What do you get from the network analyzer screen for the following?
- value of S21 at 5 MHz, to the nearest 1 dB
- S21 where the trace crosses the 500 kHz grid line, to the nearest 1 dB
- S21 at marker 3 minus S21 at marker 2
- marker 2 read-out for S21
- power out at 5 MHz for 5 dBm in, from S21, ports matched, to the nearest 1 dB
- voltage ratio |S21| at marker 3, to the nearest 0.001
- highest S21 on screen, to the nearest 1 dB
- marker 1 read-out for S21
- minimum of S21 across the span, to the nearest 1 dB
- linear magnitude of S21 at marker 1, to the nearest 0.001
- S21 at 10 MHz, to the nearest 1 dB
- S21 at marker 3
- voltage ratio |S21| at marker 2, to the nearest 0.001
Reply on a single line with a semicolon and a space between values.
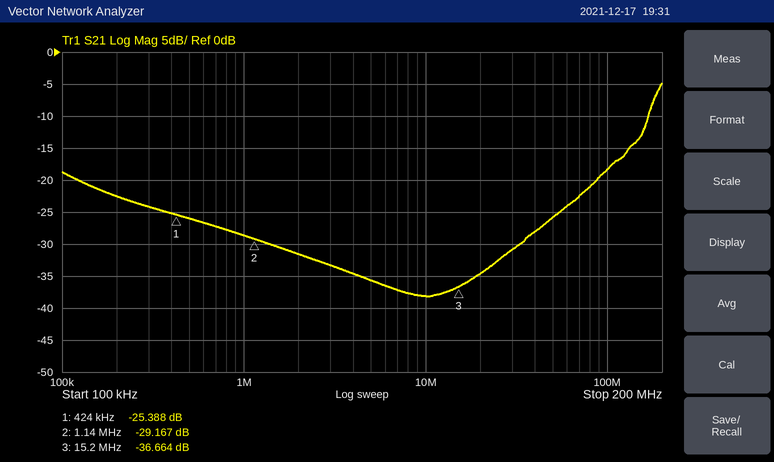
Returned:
-36 dB; -26 dB; -7.497 dB; -29.167 dB; -31 dBm; 0.015; -5 dB; -25.388 dB; -38 dB; 0.054; -38 dB; -36.664 dB; 0.035
